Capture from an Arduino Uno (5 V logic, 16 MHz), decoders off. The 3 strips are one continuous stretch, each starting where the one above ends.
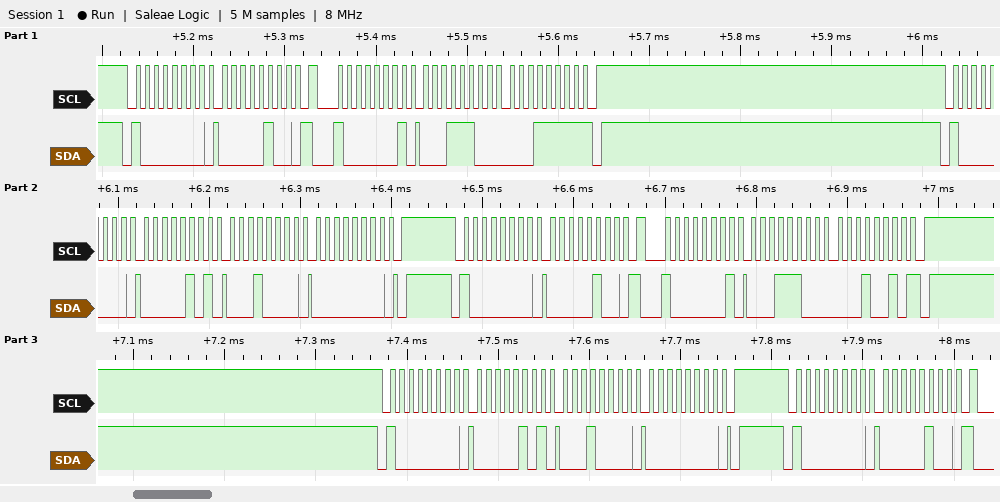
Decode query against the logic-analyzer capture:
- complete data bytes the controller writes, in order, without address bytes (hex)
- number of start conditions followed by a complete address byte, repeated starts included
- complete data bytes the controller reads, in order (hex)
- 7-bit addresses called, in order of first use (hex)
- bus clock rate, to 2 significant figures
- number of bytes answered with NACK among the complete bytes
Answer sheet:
04 05 10 00 04 05 10 00 04
7
1C 1F 1C 12
0x40
100 kHz
2
